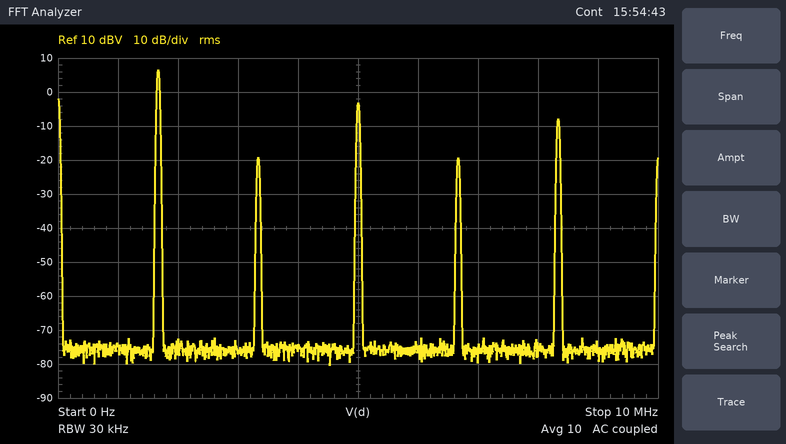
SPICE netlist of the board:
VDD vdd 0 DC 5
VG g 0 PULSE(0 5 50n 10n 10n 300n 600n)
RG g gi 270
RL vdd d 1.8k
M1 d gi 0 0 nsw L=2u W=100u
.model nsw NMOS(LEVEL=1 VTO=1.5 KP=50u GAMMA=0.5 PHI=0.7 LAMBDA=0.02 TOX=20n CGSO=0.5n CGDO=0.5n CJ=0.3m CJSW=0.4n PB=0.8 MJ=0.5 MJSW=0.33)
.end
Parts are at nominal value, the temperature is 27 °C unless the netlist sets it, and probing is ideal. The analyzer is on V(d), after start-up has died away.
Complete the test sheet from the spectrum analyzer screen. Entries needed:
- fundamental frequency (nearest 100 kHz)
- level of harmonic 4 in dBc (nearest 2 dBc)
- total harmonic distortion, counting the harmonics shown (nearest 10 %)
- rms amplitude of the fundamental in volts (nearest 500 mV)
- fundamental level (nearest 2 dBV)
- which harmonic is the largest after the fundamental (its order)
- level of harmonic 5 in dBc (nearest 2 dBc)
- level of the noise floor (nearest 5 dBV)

1.7 MHz
-26 dBc
40 %
2.0 V
6 dBV
3
-14 dBc
-75 dBV
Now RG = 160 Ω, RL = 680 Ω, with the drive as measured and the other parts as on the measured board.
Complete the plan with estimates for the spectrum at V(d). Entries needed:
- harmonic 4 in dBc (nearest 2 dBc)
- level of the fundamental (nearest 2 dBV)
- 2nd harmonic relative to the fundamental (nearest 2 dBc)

-28 dBc
6 dBV
-28 dBc
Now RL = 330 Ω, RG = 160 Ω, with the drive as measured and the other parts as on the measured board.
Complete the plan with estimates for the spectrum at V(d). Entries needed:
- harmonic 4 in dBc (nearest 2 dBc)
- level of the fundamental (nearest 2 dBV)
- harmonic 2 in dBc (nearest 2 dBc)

-30 dBc
4 dBV
-30 dBc
